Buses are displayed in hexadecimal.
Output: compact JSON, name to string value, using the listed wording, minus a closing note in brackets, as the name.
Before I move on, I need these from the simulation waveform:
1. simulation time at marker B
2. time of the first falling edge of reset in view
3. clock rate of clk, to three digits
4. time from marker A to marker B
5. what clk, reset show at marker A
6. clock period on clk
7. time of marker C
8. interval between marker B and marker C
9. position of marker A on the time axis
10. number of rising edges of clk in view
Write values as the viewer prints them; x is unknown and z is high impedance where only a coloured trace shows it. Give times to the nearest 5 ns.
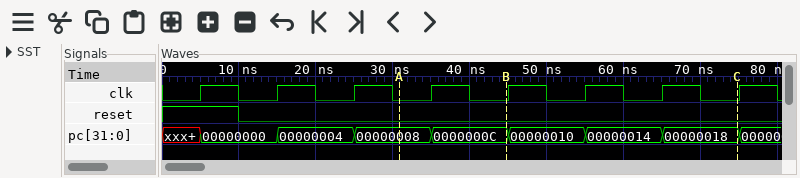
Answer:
{"simulation time at marker B": "45 ns", "time of the first falling edge of reset in view": "10 ns", "clock rate of clk, to three digits": "100 MHz", "time from marker A to marker B": "15 ns", "what clk, reset show at marker A": "clk=0, reset=0", "clock period on clk": "10 ns", "time of marker C": "75 ns", "interval between marker B and marker C": "30 ns", "position of marker A on the time axis": "30 ns", "number of rising edges of clk in view": "8"}
